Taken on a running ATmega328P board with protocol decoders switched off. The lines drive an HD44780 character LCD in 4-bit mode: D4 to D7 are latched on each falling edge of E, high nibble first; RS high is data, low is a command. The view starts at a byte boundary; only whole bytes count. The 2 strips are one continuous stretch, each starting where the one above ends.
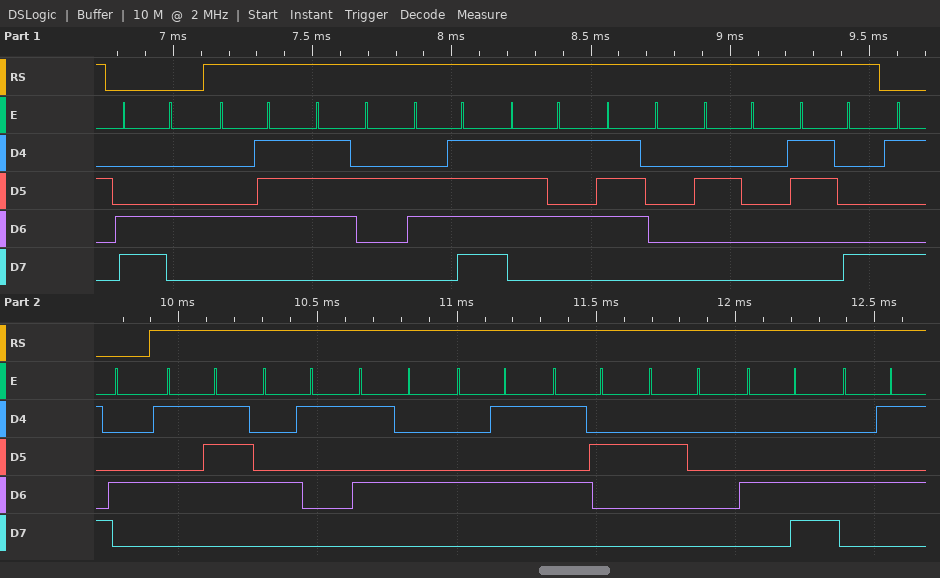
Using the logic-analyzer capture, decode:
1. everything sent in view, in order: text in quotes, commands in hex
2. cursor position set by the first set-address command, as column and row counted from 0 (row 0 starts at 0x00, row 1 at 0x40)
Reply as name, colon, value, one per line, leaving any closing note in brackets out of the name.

everything sent in view, in order: text in quotes, commands in hex: 0xC4 "Group 8" 0x94 "WATER LE"
cursor position set by the first set-address command, as column and row counted from 0: column 4, row 1
